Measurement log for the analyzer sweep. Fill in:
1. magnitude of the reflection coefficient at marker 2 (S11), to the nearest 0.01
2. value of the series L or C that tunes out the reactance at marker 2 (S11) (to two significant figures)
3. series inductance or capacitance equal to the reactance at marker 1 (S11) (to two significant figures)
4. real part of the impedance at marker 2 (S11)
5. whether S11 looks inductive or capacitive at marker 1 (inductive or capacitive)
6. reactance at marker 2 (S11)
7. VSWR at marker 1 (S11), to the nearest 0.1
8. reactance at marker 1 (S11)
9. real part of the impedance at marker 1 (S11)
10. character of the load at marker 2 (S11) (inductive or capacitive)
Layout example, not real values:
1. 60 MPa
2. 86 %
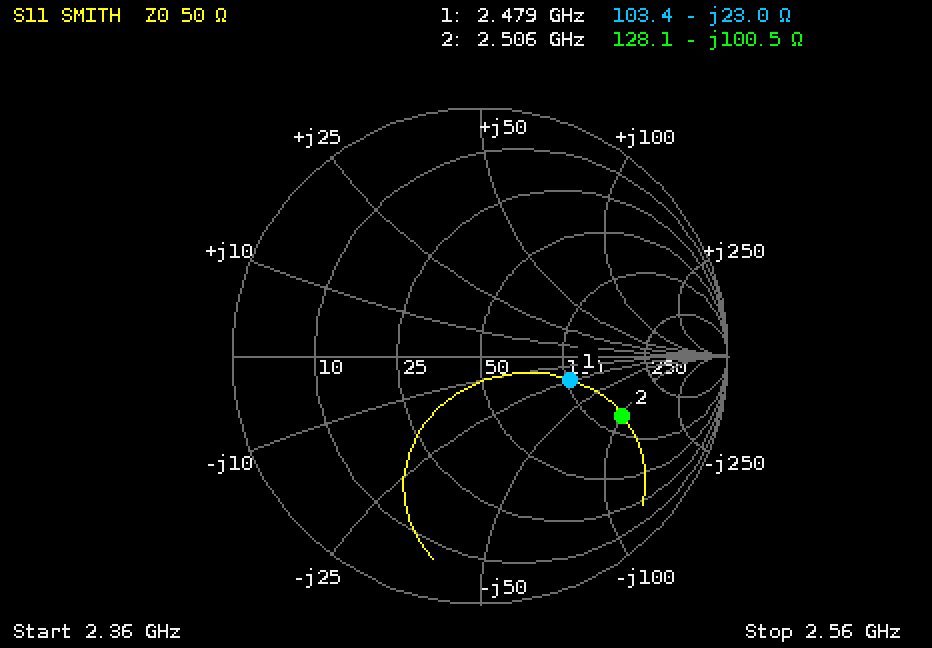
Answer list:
1. 0.62
2. 6.4 nH
3. 2.8 pF
4. 128.1 Ω
5. capacitive
6. -100.5 Ω
7. 2.2
8. -23.0 Ω
9. 103.4 Ω
10. capacitive
